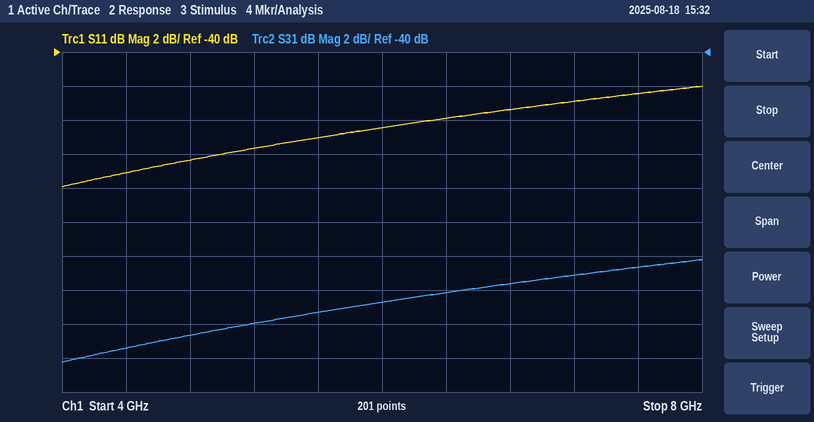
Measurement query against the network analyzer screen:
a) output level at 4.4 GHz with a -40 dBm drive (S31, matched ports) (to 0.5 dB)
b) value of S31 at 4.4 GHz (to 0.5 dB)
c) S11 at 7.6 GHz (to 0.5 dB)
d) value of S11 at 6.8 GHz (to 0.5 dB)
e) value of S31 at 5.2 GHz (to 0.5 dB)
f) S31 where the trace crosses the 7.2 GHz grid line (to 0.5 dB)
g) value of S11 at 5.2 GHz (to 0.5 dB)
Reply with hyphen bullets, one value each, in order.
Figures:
- -97.5 dBm
- -57.5 dB
- -42.5 dB
- -43.5 dB
- -56.0 dB
- -53.0 dB
- -45.5 dB
